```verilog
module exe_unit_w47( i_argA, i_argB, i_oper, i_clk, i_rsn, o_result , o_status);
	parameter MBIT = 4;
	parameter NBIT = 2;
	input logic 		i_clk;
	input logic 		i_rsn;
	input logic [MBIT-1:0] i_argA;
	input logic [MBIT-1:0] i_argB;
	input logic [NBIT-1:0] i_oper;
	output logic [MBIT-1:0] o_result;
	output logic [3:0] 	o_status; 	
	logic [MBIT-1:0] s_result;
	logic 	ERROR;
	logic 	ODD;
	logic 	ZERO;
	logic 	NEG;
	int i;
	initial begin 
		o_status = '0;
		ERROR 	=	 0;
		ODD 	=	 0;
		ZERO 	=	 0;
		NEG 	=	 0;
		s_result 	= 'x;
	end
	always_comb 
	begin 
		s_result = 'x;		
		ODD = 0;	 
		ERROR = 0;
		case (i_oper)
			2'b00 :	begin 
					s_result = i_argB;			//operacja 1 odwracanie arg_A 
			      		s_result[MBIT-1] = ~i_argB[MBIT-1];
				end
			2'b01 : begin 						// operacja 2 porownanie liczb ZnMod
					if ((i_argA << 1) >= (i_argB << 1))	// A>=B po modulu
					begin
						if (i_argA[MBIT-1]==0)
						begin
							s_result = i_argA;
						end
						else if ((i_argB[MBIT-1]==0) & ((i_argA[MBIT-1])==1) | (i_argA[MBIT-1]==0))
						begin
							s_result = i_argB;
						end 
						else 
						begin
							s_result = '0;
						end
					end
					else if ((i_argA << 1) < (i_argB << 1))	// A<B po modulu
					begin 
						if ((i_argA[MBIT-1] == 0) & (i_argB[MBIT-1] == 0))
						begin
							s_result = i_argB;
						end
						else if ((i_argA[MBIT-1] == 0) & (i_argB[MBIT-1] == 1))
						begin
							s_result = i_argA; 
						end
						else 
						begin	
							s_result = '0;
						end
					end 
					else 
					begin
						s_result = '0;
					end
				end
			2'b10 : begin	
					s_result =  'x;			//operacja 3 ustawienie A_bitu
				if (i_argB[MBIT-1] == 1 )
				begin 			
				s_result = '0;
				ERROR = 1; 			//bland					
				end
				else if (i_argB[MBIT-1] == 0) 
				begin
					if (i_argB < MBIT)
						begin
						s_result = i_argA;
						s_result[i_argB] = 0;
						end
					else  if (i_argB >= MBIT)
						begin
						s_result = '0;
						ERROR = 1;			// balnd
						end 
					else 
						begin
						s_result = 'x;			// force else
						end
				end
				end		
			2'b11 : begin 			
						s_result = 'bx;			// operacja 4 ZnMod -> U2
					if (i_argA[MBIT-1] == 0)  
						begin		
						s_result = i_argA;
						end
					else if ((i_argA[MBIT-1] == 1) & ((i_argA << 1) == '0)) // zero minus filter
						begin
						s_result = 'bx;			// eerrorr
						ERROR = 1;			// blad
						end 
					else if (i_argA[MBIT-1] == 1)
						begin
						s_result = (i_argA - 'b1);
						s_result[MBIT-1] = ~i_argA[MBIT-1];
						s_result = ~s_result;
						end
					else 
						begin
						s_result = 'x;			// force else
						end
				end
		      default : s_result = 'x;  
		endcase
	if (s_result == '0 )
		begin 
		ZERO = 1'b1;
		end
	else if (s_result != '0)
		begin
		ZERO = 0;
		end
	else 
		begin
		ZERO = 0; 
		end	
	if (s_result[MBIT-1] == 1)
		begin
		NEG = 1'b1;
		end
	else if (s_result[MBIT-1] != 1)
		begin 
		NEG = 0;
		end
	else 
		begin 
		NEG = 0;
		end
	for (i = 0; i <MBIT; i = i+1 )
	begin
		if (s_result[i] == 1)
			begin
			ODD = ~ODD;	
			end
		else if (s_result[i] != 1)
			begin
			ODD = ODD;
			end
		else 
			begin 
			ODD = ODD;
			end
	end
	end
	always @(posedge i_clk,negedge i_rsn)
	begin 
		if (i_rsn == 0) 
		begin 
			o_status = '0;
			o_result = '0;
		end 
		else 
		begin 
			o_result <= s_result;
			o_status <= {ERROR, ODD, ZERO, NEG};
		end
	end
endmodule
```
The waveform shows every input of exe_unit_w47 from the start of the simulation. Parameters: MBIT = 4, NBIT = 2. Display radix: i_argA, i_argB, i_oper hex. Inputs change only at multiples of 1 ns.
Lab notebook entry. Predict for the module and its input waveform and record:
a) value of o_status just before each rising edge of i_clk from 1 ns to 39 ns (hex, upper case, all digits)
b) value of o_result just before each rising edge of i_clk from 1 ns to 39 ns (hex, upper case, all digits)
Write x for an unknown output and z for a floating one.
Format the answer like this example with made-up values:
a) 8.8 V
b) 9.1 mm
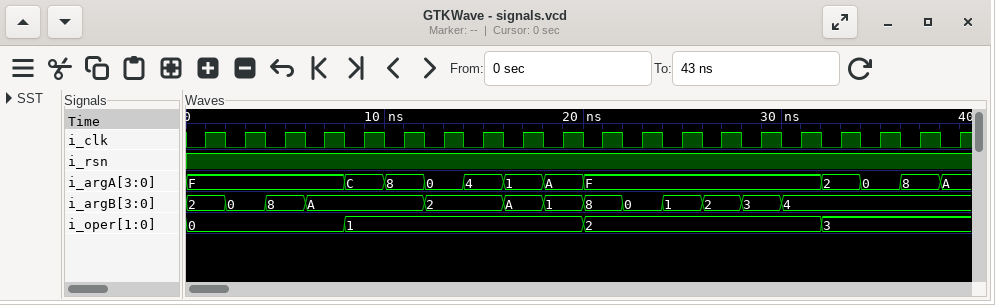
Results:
a) 0, 1, 5, 2, 4, 2, 2, 4, 4, 4, 4, A, 5, 5, 5, 4, A, 4, 2, 8
b) x, A, 8, 0, 2, 0, 0, 2, 4, 1, 1, 0, E, D, B, 7, 0, 2, 0, x
